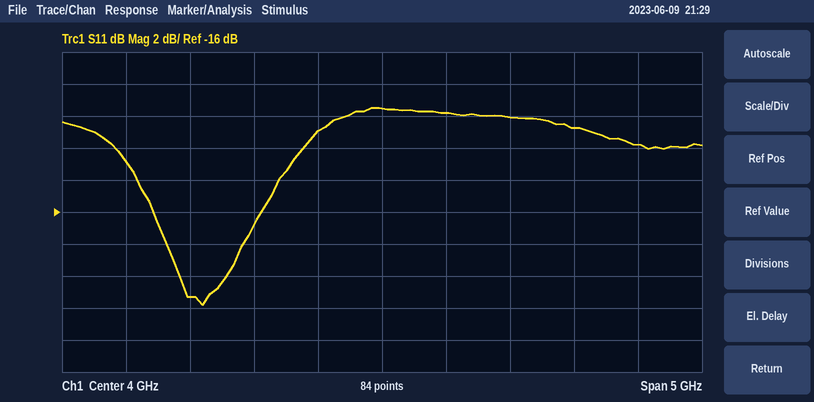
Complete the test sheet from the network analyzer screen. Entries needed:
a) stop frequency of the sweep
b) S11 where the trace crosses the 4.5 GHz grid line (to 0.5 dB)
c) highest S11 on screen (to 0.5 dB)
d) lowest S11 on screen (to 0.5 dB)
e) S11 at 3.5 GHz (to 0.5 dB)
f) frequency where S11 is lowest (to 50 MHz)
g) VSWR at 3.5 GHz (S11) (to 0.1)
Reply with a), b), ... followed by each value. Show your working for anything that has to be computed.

a) 6.5 GHz
b) -10.0 dB
c) -9.5 dB
d) -22.0 dB
e) -11.0 dB
f) 2.60 GHz
g) |Γ| = 10^(-11/20) = 0.2818; VSWR = (1 + 0.2818)/(1 − 0.2818) ≈ 1.8
